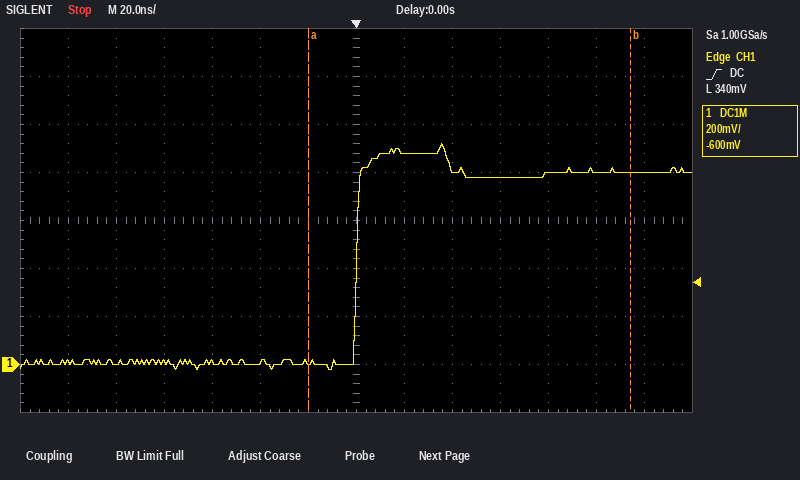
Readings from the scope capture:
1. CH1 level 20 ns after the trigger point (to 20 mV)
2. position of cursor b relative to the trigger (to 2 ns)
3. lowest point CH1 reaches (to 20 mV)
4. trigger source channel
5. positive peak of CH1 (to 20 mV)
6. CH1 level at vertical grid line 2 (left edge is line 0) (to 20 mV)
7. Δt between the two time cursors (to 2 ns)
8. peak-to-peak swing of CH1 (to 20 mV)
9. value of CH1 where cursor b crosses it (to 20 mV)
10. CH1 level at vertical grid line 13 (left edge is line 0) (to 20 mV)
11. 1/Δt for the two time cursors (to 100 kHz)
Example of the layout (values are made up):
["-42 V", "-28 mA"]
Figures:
["880 mV", "+114 ns", "-20 mV", "CH1", "920 mV", "0 mV", "134 ns", "940 mV", "800 mV", "800 mV", "7.5 MHz"]
